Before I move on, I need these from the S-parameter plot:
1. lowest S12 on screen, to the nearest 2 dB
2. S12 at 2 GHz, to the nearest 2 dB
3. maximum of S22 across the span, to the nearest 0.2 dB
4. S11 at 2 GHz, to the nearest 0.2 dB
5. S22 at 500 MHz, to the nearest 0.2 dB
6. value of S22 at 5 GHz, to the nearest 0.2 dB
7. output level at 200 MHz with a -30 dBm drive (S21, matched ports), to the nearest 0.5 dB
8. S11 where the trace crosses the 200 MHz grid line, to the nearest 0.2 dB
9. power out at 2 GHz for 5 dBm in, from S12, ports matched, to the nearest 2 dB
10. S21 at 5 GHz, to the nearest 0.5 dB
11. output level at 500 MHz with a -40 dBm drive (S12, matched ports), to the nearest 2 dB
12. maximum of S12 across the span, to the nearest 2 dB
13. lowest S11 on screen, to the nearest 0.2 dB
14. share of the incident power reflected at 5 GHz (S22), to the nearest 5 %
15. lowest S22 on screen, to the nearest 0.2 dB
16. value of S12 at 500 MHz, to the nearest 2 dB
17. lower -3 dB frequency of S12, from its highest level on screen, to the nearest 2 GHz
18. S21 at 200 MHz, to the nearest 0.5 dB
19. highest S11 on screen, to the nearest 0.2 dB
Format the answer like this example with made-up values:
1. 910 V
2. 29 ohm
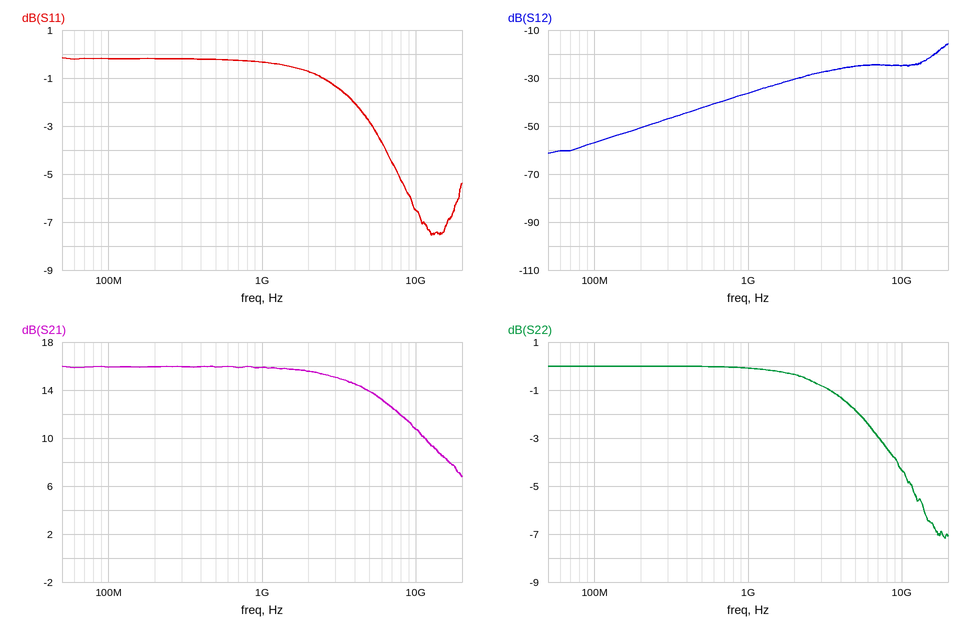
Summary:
1. -62 dB
2. -30 dB
3. 0.0 dB
4. -0.8 dB
5. 0.0 dB
6. -1.8 dB
7. -14.0 dBm
8. -0.2 dB
9. -26 dBm
10. 14.0 dB
11. -82 dBm
12. -16 dB
13. -7.6 dB
14. 65 %
15. -7.2 dB
16. -42 dB
17. 18 GHz
18. 16.0 dB
19. -0.2 dB
